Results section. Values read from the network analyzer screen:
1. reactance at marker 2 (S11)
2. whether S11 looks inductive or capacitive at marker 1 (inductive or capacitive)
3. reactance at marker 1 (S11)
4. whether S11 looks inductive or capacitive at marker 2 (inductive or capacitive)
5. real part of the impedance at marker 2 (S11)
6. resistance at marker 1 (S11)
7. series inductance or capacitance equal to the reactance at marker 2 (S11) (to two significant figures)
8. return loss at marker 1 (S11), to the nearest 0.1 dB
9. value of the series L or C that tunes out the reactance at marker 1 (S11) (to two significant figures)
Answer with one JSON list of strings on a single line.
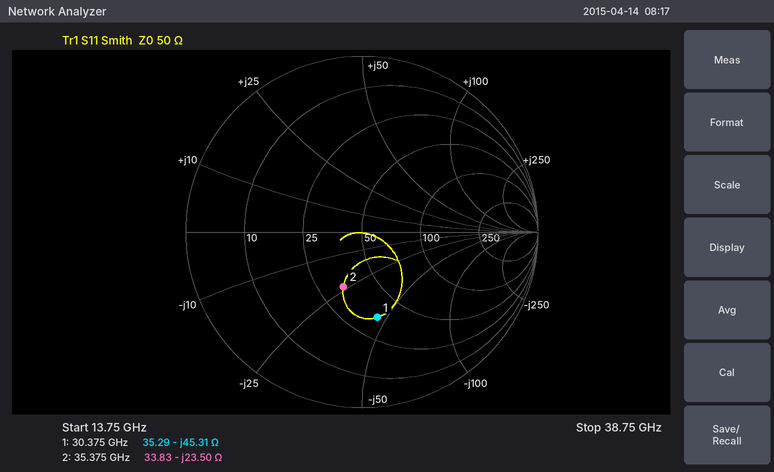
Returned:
["-23.50 Ω", "capacitive", "-45.31 Ω", "capacitive", "33.83 Ω", "35.29 Ω", "190 fF", "6.1 dB", "240 pH"]
